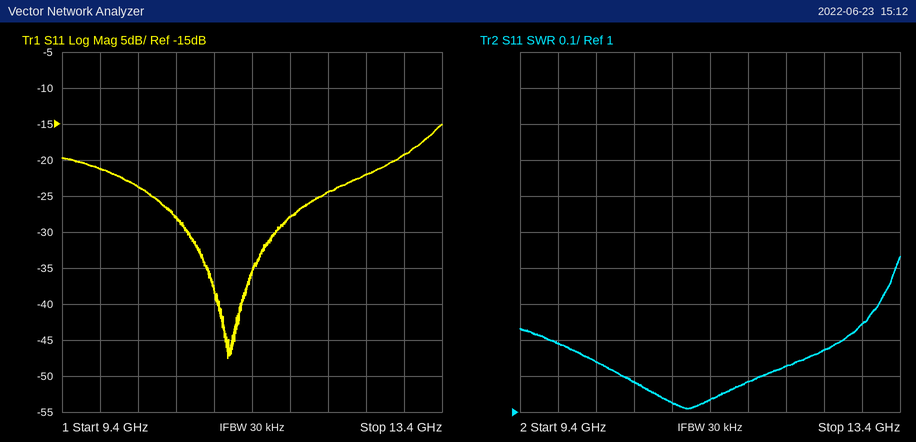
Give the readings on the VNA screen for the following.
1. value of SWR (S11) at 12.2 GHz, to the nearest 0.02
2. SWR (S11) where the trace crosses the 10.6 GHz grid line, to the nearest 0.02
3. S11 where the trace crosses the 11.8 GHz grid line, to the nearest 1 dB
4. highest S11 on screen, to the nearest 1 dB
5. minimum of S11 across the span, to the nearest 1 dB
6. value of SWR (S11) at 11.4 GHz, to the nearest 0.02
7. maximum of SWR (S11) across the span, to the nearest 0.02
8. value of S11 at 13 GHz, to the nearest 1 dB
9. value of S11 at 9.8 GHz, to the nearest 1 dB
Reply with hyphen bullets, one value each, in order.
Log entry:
- 1.12
- 1.08
- -28 dB
- -15 dB
- -48 dB
- 1.04
- 1.44
- -19 dB
- -21 dB
